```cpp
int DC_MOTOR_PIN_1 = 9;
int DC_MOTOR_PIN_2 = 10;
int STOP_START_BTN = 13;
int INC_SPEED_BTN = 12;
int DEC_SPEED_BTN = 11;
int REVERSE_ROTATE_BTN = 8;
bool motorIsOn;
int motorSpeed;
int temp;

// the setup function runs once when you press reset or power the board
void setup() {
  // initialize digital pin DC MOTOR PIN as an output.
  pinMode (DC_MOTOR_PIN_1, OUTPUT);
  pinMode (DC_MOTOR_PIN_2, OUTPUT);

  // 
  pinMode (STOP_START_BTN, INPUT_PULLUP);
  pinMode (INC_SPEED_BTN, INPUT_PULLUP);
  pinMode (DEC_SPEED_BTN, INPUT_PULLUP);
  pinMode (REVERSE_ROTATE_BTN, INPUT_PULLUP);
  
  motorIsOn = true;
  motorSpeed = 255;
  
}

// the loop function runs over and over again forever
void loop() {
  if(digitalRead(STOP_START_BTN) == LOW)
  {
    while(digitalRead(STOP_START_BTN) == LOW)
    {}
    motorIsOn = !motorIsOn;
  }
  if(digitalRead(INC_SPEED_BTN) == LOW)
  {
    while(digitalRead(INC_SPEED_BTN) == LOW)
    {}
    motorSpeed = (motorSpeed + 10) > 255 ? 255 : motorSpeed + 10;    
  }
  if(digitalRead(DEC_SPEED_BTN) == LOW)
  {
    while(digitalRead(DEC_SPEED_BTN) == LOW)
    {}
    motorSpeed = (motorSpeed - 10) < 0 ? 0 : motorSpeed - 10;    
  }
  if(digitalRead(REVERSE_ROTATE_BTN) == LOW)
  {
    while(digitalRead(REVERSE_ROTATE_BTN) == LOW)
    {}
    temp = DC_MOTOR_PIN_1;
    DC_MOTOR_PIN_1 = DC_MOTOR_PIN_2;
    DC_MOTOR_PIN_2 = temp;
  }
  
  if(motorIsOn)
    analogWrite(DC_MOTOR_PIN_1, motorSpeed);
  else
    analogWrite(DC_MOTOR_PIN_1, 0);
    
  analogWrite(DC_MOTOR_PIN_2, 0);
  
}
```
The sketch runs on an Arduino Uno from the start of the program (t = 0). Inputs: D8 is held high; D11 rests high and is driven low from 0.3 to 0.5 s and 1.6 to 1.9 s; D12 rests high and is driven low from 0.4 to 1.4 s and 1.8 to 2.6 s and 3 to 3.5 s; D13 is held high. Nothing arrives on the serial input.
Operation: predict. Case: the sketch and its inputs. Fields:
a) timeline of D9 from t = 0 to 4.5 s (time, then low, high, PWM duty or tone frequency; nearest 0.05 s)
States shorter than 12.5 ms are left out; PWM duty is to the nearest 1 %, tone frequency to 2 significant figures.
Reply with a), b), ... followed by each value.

a) 0 s high; 0.5 s PWM 96 %; 1.4 s high; 1.9 s PWM 96 %; 2.6 s high
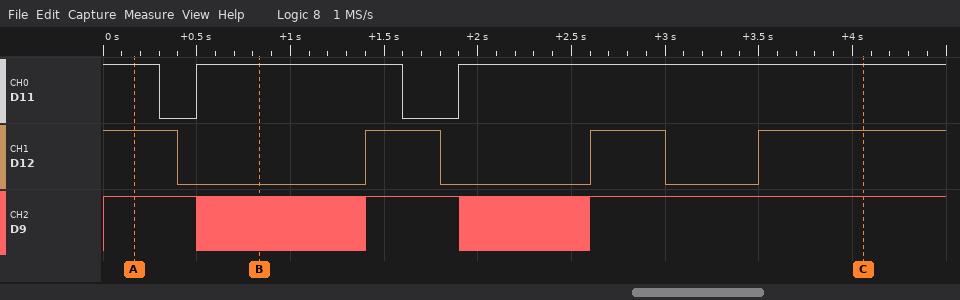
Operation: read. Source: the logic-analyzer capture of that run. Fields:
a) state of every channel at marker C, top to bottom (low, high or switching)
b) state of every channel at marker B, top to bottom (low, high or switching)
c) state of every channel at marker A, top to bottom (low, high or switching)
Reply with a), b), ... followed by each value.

a) D11 high, D12 high, D9 high
b) D11 high, D12 low, D9 switching
c) D11 high, D12 high, D9 high
